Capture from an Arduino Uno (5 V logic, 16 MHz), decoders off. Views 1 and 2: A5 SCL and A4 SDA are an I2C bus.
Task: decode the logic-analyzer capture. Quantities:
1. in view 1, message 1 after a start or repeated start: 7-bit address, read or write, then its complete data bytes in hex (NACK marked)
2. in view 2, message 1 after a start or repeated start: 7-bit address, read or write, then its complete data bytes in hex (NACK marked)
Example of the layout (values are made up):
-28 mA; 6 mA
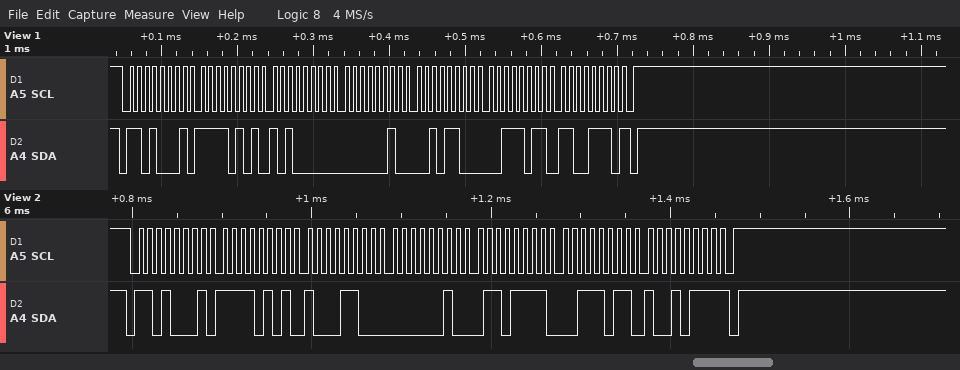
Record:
0x68 read: F5 A0 02 2C 3B CE NACK; 0x68 read: F5 8C 02 6F 3B 97 NACK
